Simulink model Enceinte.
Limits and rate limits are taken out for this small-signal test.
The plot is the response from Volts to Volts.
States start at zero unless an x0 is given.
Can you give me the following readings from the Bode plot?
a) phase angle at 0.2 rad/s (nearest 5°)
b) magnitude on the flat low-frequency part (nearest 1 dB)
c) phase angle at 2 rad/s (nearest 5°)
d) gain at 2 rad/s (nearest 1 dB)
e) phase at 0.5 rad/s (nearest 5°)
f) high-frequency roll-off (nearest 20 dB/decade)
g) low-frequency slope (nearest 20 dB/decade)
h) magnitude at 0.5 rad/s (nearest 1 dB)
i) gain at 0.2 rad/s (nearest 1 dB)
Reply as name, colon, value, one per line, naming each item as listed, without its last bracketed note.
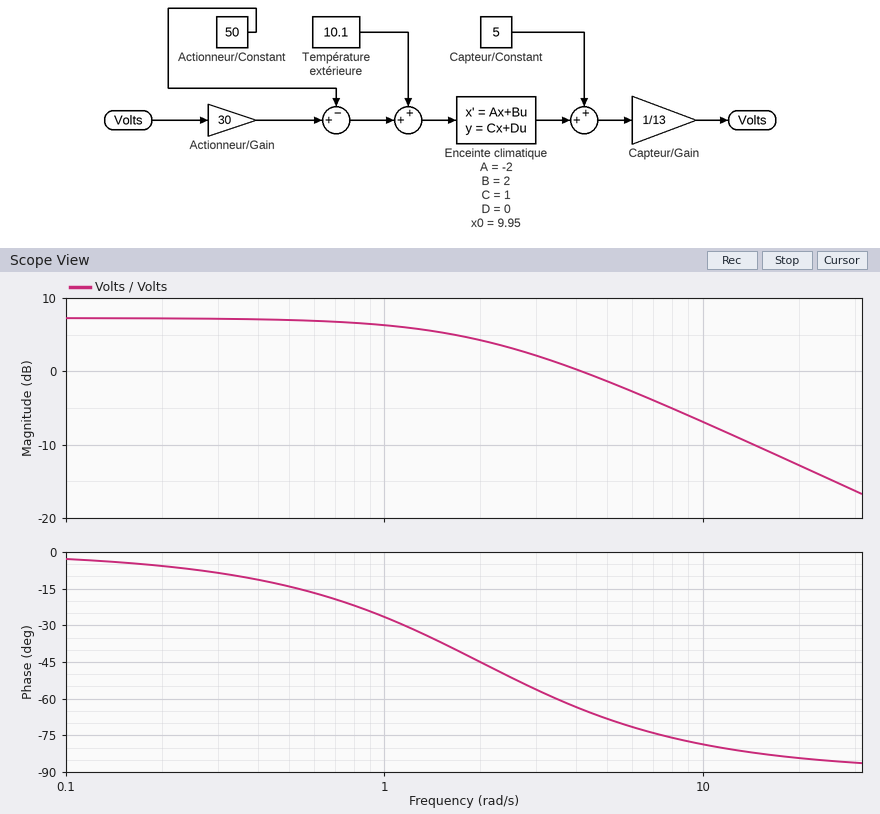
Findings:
phase angle at 0.2 rad/s: -5°
magnitude on the flat low-frequency part: 7 dB
phase angle at 2 rad/s: -45°
gain at 2 rad/s: 4 dB
phase at 0.5 rad/s: -15°
high-frequency roll-off: -20 dB/decade
low-frequency slope: 0 dB/decade
magnitude at 0.5 rad/s: 7 dB
gain at 0.2 rad/s: 7 dB
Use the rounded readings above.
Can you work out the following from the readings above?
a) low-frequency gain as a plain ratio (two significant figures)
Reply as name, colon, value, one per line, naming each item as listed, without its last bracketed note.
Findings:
low-frequency gain as a plain ratio: 2.2
